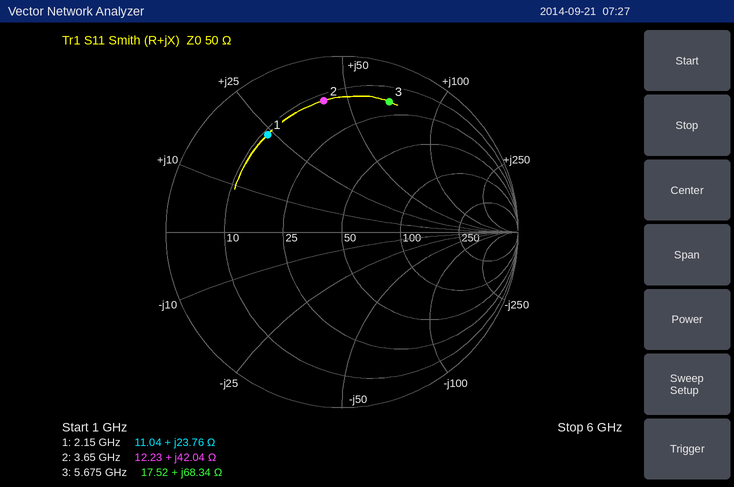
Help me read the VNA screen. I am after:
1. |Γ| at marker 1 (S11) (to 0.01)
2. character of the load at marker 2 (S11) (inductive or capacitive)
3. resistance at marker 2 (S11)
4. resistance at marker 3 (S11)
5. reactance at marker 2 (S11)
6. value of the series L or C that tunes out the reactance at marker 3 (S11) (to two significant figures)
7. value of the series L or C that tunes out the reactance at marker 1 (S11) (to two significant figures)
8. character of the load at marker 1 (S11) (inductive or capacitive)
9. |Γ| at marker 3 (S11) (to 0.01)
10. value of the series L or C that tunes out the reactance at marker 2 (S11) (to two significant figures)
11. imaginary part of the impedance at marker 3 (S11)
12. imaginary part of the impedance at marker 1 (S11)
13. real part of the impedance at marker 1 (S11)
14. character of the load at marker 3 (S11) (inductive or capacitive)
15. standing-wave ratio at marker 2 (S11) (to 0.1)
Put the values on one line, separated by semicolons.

0.70; inductive; 12.23 Ω; 17.52 Ω; +42.04 Ω; 410 fF; 3.1 pF; inductive; 0.79; 1.0 pF; +68.34 Ω; +23.76 Ω; 11.04 Ω; inductive; 7.1
